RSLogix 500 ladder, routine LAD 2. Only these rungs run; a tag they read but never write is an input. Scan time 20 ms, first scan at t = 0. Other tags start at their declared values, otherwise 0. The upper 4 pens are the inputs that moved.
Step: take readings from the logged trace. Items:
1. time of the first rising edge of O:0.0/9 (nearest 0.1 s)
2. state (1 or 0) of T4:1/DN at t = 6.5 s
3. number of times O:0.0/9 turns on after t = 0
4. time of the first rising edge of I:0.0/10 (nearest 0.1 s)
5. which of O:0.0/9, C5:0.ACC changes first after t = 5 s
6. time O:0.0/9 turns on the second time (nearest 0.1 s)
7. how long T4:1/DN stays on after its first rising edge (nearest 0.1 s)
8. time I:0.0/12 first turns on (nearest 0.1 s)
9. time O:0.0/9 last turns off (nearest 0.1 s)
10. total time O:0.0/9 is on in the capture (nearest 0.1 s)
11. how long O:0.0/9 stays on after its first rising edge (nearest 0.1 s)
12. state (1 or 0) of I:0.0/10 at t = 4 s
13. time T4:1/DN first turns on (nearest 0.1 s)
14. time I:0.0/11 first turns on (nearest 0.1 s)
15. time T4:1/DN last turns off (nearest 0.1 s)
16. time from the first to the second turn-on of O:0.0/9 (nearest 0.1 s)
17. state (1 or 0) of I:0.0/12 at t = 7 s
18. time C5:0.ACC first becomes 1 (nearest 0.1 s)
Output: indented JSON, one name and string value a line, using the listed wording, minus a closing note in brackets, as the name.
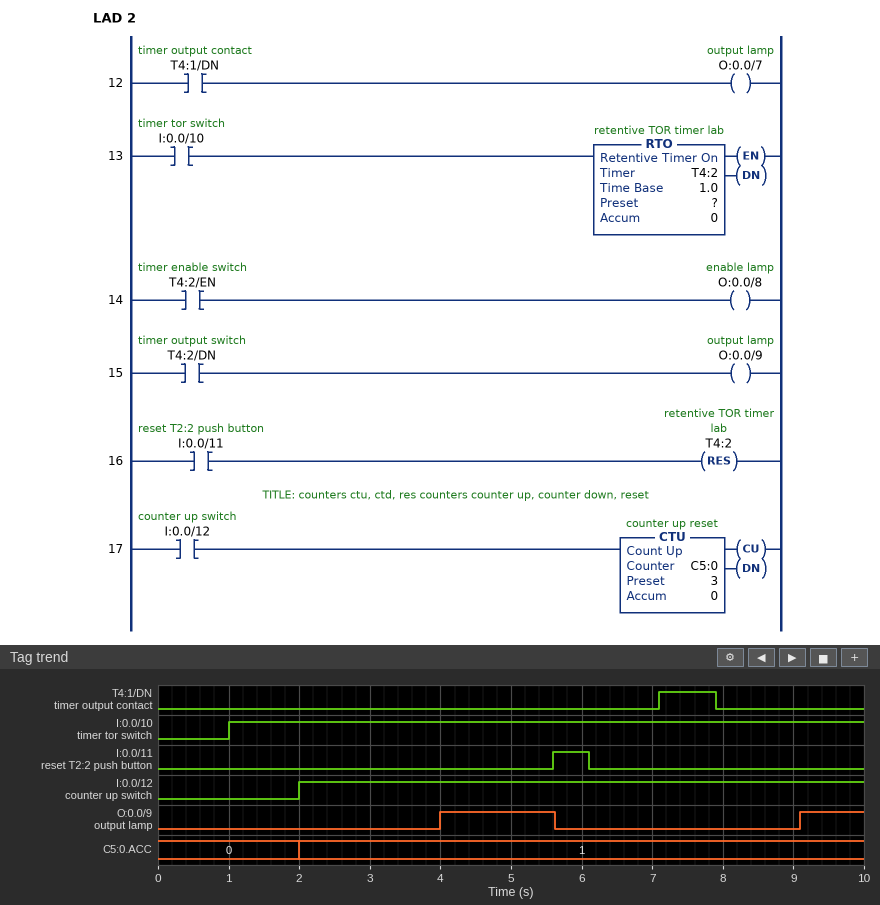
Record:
{
  "time of the first rising edge of O:0.0/9": "4.0 s",
  "state (1 or 0) of T4:1/DN at t = 6.5 s": "0",
  "number of times O:0.0/9 turns on after t = 0": "2",
  "time of the first rising edge of I:0.0/10": "1.0 s",
  "which of O:0.0/9, C5:0.ACC changes first after t = 5 s": "O:0.0/9",
  "time O:0.0/9 turns on the second time": "9.1 s",
  "how long T4:1/DN stays on after its first rising edge": "0.8 s",
  "time I:0.0/12 first turns on": "2.0 s",
  "time O:0.0/9 last turns off": "5.6 s",
  "total time O:0.0/9 is on in the capture": "2.5 s",
  "how long O:0.0/9 stays on after its first rising edge": "1.6 s",
  "state (1 or 0) of I:0.0/10 at t = 4 s": "1",
  "time T4:1/DN first turns on": "7.1 s",
  "time I:0.0/11 first turns on": "5.6 s",
  "time T4:1/DN last turns off": "7.9 s",
  "time from the first to the second turn-on of O:0.0/9": "5.1 s",
  "state (1 or 0) of I:0.0/12 at t = 7 s": "1",
  "time C5:0.ACC first becomes 1": "2.0 s"
}
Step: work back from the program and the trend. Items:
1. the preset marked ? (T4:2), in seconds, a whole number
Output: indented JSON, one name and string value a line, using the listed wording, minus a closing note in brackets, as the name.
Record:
{
  "the preset marked ? (T4:2), in seconds, a whole number": "3 s"
}
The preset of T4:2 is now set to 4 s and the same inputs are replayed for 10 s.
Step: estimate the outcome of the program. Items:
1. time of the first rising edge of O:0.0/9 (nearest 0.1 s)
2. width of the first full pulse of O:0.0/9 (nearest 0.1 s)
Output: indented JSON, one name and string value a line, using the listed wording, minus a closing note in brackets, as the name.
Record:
{
  "time of the first rising edge of O:0.0/9": "5.0 s",
  "width of the first full pulse of O:0.0/9": "0.6 s"
}
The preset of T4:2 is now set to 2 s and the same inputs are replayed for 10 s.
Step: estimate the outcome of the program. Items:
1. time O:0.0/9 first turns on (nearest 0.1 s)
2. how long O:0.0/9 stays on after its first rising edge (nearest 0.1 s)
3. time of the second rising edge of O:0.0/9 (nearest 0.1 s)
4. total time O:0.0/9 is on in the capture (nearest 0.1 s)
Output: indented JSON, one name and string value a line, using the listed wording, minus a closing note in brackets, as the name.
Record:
{
  "time O:0.0/9 first turns on": "3.0 s",
  "how long O:0.0/9 stays on after its first rising edge": "2.6 s",
  "time of the second rising edge of O:0.0/9": "8.1 s",
  "total time O:0.0/9 is on in the capture": "4.5 s"
}
